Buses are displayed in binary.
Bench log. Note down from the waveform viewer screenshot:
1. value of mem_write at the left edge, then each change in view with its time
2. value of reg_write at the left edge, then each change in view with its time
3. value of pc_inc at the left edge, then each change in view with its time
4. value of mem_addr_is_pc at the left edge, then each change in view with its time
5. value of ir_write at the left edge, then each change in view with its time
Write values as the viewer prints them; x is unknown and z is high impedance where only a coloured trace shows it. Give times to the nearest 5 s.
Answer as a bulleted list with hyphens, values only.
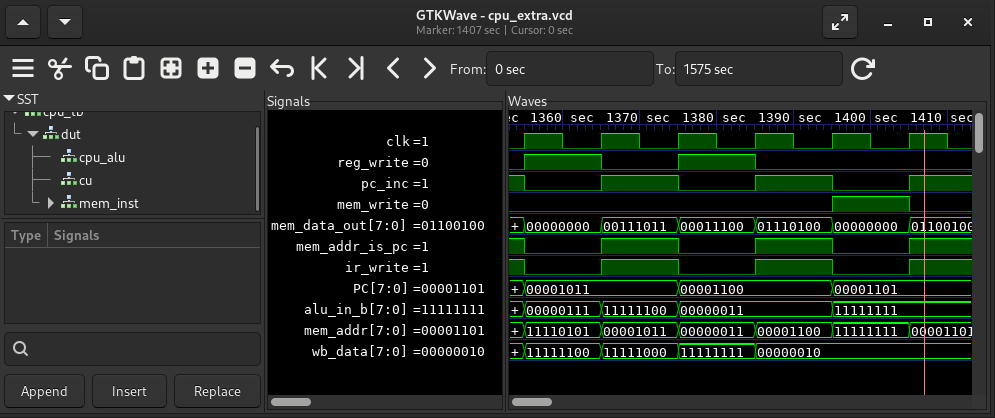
- 0, 1 at 1395 s, 0 at 1405 s
- 0, 1 at 1355 s, 0 at 1365 s, 1 at 1375 s, 0 at 1385 s
- 1, 0 at 1355 s, 1 at 1365 s, 0 at 1375 s, 1 at 1385 s, 0 at 1395 s, 1 at 1405 s
- 1, 0 at 1355 s, 1 at 1365 s, 0 at 1375 s, 1 at 1385 s, 0 at 1395 s, 1 at 1405 s
- 1, 0 at 1355 s, 1 at 1365 s, 0 at 1375 s, 1 at 1385 s, 0 at 1395 s, 1 at 1405 s
